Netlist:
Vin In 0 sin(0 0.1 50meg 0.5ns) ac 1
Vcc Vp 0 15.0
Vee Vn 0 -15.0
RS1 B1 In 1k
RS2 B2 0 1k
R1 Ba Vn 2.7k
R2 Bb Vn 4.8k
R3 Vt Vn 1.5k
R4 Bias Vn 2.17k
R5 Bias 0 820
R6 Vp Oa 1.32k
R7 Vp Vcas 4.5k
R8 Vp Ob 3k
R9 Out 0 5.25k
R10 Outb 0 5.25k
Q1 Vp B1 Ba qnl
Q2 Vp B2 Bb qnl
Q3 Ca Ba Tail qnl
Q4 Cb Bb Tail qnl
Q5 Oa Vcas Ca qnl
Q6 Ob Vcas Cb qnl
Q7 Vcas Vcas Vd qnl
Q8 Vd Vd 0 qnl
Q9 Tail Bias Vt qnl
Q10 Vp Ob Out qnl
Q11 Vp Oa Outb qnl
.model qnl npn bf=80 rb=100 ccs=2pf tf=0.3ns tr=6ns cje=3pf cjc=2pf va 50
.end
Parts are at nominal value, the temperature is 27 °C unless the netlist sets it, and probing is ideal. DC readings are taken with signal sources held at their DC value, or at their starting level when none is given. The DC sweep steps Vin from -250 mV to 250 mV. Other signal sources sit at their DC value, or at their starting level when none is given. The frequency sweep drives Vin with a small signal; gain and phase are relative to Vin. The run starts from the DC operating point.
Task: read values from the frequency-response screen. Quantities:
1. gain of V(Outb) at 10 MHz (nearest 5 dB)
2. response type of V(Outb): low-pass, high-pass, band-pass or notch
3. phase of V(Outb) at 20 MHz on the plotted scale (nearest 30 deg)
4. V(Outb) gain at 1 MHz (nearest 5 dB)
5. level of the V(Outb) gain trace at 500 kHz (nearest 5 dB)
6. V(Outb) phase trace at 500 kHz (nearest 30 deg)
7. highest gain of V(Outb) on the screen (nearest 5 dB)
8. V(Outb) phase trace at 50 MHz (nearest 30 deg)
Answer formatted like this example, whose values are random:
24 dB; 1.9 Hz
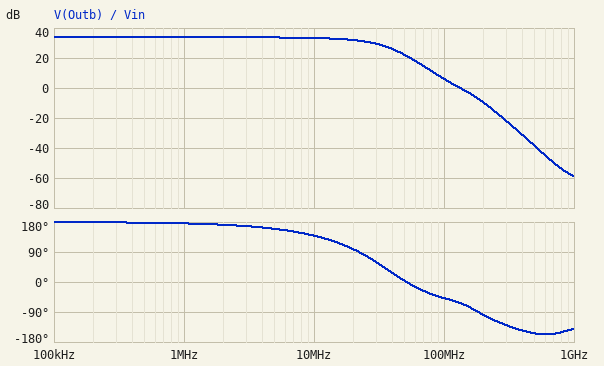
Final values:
35 dB; low-pass; 90 deg; 35 dB; 35 dB; 180 deg; 35 dB; 0 deg
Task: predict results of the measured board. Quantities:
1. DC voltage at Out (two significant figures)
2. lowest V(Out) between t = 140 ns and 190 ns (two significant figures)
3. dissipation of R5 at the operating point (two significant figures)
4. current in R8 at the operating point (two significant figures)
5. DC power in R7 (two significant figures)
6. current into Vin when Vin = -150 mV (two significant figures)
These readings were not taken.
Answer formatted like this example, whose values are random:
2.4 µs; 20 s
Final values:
150 mV; 65 mV; 21 mW; 4.7 mA; 40 mW; -49 µA
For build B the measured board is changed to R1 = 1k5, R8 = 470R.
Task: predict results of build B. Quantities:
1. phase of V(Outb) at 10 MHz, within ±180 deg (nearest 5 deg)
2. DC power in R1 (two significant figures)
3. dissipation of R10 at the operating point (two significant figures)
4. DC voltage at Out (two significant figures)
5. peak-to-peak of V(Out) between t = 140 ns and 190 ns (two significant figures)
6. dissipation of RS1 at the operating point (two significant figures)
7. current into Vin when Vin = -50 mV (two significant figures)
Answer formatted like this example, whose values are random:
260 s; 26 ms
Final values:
145 deg; 130 mW; 37 mW; 11 V; 920 mV; 8.0 µW; -89 µA
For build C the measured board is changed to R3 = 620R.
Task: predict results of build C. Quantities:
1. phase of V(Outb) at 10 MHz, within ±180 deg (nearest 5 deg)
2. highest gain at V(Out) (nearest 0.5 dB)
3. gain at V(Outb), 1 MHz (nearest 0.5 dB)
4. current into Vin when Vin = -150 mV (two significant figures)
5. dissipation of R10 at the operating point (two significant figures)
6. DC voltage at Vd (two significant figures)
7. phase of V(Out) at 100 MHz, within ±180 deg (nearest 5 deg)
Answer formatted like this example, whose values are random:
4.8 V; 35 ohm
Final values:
160 deg; 5.0 dB; 21.0 dB; -50 µA; 6.2 mW; -140 mV; -130 deg
